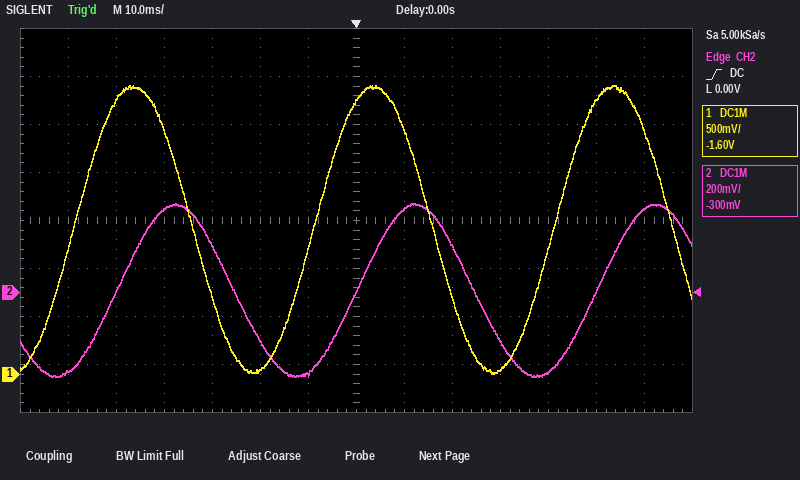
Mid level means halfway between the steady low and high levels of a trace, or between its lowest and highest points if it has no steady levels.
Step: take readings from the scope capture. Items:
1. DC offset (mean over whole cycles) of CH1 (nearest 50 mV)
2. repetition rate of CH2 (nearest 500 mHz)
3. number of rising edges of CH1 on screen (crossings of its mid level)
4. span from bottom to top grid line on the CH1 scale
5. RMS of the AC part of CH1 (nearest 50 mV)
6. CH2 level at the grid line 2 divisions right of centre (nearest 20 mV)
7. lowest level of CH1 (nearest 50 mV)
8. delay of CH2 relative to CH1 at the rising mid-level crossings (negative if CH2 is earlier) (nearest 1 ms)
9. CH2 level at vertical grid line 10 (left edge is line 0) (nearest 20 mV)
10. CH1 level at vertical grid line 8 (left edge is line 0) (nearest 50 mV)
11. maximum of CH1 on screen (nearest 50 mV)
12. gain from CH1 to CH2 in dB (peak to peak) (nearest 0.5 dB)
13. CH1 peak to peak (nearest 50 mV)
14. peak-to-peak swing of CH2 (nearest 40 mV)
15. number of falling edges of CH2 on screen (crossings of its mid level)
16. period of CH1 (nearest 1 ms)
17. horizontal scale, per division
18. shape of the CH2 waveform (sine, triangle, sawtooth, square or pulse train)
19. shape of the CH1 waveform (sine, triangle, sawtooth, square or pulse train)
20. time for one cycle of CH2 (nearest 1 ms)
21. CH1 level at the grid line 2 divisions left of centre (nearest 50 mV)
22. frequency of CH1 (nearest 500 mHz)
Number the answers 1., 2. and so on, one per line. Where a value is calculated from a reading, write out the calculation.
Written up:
1. (3.00 V + (0 mV)) / 2 ≈ 1.50 V
2. 1 / 50 ms ≈ 20.0 Hz
3. 3
4. 4 V
5. 3.00 V / (2√2) ≈ 1.06 V, so 1.05 V to the nearest 50 mV
6. 200 mV
7. 0 mV
8. +9 ms
9. -200 mV
10. 2.55 V
11. 3.00 V
12. 20 log10(720 mV / 3.00 V) ≈ -12.4 dB, so -12.5 dB to the nearest 0.5 dB
13. 3.00 V − (0 mV) = 3.00 V
14. 720 mV
15. 2
16. 50 ms
17. 10 ms
18. sine
19. sine
20. 50 ms
21. 50 mV
22. 1 / 50 ms ≈ 20.0 Hz
